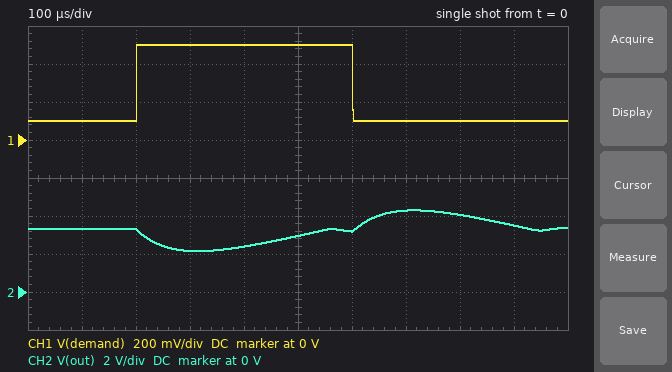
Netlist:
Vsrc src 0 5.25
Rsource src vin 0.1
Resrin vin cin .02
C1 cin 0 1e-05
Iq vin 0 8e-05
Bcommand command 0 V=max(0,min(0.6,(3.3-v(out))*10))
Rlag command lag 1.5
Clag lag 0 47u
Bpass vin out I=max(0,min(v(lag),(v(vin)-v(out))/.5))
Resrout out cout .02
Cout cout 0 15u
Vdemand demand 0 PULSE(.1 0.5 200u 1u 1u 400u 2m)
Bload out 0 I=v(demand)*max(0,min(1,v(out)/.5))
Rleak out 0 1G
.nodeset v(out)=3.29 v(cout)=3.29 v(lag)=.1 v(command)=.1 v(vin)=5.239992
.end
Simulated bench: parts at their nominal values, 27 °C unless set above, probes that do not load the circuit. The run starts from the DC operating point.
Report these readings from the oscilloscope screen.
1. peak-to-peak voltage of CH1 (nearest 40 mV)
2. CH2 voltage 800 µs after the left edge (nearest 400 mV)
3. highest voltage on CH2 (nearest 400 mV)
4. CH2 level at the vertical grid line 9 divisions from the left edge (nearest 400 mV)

400 mV
4.0 V
4.4 V
3.6 V
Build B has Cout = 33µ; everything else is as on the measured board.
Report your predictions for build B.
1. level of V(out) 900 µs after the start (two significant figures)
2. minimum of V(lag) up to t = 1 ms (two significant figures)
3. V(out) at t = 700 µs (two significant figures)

3.3 V
5.9 mV
3.7 V
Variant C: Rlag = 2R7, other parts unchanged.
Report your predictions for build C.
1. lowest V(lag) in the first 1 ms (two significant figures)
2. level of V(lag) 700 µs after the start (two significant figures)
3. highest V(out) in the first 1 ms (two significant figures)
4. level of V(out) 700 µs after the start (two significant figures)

35 mV
380 mV
5.2 V
4.7 V
